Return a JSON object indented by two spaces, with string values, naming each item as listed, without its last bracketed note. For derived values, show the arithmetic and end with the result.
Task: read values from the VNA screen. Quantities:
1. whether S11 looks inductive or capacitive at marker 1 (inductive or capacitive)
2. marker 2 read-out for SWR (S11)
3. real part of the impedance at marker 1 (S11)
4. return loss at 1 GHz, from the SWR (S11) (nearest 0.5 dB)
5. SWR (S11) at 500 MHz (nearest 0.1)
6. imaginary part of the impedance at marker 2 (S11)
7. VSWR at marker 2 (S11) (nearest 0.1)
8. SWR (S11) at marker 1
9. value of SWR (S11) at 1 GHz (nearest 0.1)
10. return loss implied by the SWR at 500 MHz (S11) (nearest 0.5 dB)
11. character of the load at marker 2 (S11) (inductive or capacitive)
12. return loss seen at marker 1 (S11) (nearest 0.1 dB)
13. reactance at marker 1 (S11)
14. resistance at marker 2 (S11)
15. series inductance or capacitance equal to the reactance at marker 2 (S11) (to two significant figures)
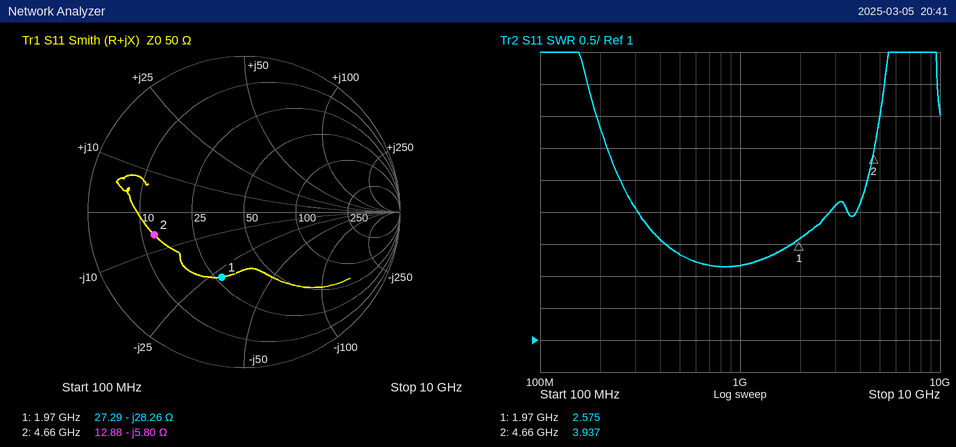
{
  "whether S11 looks inductive or capacitive at marker 1": "capacitive",
  "marker 2 read-out for SWR": "3.937",
  "real part of the impedance at marker 1": "27.29 Ω",
  "return loss at 1 GHz, from the SWR (S11)": "−20 log10((2.2 − 1)/(2.2 + 1)) ≈ 8.5 dB",
  "SWR (S11) at 500 MHz": "2.3",
  "imaginary part of the impedance at marker 2": "-5.80 Ω",
  "VSWR at marker 2 (S11)": "3.9",
  "SWR (S11) at marker 1": "2.575",
  "value of SWR (S11) at 1 GHz": "2.2",
  "return loss implied by the SWR at 500 MHz (S11)": "−20 log10((2.3 − 1)/(2.3 + 1)) ≈ 8.09 dB, so 8.0 dB to the nearest 0.5 dB",
  "character of the load at marker 2 (S11)": "capacitive",
  "return loss seen at marker 1 (S11)": "7.1 dB",
  "reactance at marker 1": "-28.26 Ω",
  "resistance at marker 2": "12.88 Ω",
  "series inductance or capacitance equal to the reactance at marker 2 (S11)": "C = 1/(2π × 4.66 GHz × 5.8 Ω) ≈ 5.9 pF"
}
